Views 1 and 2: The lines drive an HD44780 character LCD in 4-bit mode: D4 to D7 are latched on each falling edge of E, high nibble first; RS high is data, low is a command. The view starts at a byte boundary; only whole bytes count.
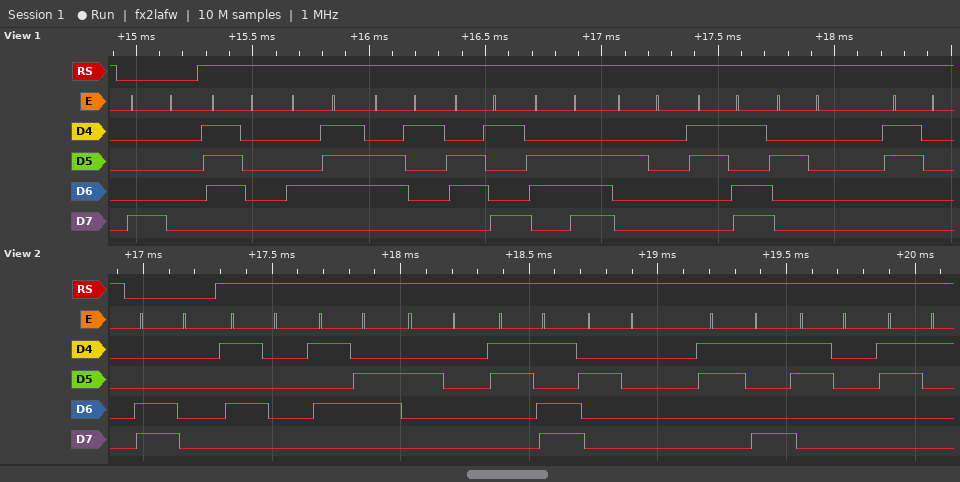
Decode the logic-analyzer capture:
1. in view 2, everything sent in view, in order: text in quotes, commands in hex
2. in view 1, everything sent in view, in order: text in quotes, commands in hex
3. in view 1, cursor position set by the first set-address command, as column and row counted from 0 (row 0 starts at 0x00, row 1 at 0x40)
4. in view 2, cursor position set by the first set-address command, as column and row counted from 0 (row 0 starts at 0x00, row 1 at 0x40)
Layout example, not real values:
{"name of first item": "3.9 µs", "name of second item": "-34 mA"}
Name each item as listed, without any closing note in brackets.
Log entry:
{"in view 2, everything sent in view, in order: text in quotes, commands in hex": "0xC0 \"PV = 901\"", "in view 1, everything sent in view, in order: text in quotes, commands in hex": "0x80 \"pGain = 0\"", "in view 1, cursor position set by the first set-address command, as column and row counted from 0": "column 0, row 0", "in view 2, cursor position set by the first set-address command, as column and row counted from 0": "column 0, row 1"}
